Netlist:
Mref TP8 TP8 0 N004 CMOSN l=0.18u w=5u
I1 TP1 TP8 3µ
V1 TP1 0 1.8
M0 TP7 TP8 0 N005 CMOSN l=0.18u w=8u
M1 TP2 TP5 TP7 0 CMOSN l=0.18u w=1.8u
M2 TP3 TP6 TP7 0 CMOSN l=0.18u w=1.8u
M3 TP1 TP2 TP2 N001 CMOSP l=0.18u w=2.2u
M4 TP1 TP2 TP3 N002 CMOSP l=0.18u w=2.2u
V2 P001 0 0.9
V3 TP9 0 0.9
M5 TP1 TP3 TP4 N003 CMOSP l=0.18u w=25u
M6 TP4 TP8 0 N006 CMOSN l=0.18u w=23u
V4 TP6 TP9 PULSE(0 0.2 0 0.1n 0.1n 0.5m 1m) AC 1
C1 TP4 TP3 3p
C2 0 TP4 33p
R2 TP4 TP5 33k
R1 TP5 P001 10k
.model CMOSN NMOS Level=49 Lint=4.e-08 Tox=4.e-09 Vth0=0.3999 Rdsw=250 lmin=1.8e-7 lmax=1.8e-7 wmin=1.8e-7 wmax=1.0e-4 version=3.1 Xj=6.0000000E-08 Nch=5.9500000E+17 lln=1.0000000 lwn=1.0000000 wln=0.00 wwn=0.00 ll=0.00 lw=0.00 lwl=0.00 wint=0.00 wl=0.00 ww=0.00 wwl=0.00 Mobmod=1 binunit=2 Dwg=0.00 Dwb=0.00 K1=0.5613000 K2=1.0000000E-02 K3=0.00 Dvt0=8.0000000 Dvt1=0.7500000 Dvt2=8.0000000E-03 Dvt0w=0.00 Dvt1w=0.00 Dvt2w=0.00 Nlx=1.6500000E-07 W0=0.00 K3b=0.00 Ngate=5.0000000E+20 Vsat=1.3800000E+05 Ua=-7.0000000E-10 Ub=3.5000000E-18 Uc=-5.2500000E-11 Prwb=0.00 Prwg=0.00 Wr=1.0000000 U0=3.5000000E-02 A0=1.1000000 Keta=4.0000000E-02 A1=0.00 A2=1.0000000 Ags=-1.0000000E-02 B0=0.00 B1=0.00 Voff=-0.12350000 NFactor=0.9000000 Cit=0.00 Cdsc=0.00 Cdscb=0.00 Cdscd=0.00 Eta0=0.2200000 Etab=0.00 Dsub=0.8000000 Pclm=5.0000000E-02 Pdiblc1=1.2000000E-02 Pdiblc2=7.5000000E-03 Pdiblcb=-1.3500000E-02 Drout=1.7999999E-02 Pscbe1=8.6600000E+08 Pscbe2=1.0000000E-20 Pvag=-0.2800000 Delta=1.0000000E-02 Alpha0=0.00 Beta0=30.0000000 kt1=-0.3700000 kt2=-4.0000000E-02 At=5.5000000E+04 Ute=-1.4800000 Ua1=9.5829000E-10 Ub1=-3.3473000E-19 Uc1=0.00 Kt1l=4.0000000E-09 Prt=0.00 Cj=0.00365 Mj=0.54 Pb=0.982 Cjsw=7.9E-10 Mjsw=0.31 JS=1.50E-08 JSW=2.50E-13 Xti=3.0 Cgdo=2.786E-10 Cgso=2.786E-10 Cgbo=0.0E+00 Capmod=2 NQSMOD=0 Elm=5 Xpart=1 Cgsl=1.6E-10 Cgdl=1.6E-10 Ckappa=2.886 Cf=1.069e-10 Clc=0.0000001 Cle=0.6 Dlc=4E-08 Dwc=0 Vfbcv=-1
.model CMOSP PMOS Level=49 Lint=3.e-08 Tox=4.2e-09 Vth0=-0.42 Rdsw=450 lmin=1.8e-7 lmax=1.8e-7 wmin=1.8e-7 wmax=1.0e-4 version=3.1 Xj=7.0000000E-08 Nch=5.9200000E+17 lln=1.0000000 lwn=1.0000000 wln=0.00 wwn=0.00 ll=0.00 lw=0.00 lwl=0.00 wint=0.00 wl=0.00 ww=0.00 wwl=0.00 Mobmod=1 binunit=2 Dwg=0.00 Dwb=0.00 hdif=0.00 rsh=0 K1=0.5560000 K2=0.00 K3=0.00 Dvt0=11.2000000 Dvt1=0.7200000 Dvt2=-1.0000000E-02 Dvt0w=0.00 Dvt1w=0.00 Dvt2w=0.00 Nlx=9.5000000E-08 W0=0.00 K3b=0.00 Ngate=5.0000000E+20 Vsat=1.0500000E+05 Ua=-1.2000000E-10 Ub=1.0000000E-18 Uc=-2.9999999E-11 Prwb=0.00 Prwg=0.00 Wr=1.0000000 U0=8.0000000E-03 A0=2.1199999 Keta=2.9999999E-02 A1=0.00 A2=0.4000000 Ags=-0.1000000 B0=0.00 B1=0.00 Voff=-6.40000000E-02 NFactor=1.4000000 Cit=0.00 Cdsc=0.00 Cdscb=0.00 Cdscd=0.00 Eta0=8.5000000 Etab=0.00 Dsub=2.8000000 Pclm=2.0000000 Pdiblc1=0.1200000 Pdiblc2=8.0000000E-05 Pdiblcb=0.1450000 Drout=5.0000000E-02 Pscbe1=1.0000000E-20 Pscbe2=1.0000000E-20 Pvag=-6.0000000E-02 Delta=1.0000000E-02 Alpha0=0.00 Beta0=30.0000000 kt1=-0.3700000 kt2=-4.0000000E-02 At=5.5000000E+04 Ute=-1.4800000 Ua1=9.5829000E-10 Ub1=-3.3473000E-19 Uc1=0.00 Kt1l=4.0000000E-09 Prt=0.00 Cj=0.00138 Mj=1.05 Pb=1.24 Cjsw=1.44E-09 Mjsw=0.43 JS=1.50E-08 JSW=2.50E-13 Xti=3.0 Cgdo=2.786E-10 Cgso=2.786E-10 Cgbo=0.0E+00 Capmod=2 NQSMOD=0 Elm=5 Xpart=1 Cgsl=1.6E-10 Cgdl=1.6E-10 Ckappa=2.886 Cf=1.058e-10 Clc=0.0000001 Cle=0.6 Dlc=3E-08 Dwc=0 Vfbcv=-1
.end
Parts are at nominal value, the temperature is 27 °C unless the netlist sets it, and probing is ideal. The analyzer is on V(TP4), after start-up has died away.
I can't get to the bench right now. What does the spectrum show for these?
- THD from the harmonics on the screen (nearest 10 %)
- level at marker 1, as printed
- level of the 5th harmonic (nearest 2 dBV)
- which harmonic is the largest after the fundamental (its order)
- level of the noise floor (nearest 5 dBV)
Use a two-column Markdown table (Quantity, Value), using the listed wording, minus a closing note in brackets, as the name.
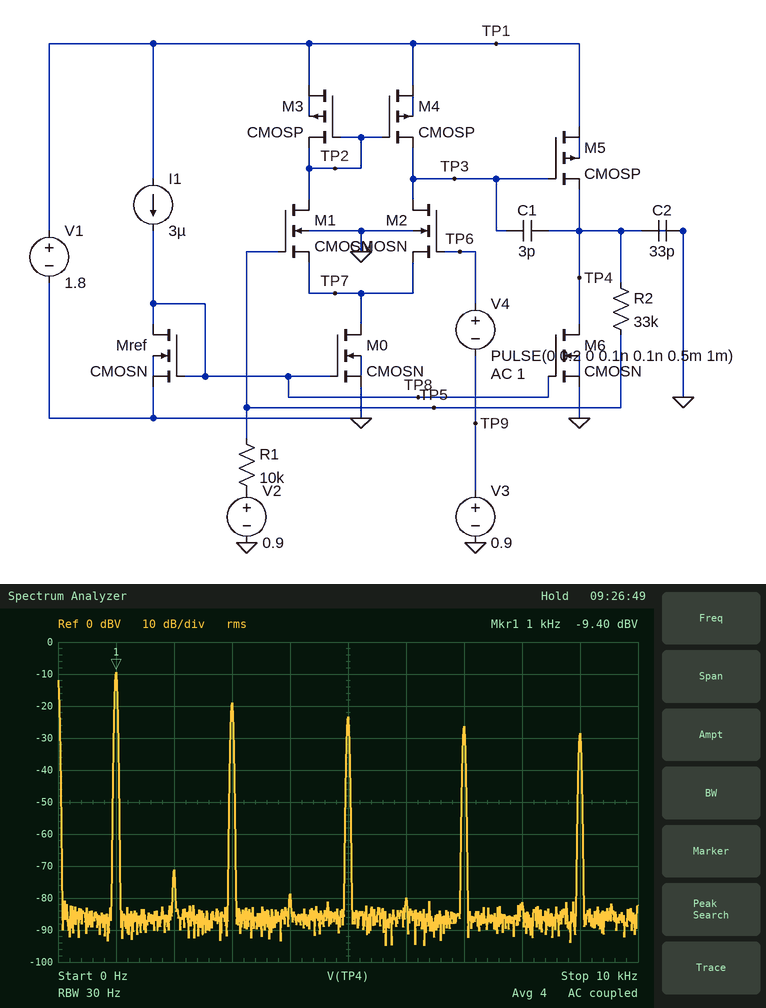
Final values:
| Quantity | Value |
|---|---|
| THD from the harmonics on the screen | 40 % |
| level at marker 1, as printed | -9.40 dBV |
| level of the 5th harmonic | -24 dBV |
| which harmonic is the largest after the fundamental | 3 |
| level of the noise floor | -85 dBV |
